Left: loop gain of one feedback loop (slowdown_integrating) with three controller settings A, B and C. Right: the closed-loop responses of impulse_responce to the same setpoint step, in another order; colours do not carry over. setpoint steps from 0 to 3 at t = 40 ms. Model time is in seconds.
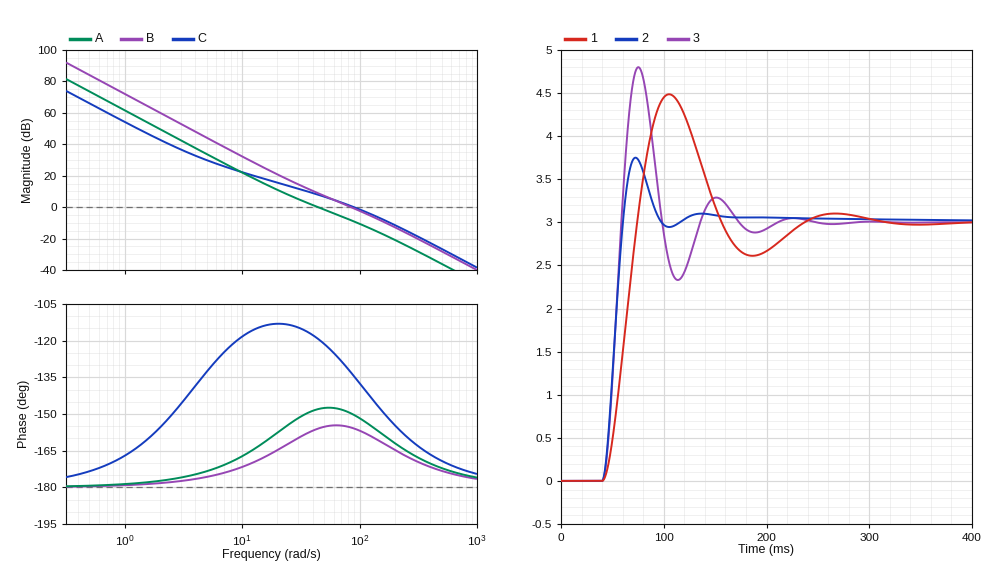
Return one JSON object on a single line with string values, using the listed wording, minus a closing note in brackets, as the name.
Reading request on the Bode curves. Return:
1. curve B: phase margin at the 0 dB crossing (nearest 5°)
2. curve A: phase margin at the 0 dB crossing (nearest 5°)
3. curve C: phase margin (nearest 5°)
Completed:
{"curve B: phase margin at the 0 dB crossing": "25°", "curve A: phase margin at the 0 dB crossing": "30°", "curve C: phase margin": "45°"}
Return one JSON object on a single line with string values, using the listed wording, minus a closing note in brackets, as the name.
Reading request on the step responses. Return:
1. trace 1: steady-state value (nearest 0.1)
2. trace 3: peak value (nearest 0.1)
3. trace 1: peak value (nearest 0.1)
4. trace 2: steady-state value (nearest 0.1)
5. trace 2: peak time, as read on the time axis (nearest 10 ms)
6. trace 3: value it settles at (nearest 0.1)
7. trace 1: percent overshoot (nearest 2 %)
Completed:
{"trace 1: steady-state value": "3.0", "trace 3: peak value": "4.8", "trace 1: peak value": "4.5", "trace 2: steady-state value": "3.0", "trace 2: peak time, as read on the time axis": "70 ms", "trace 3: value it settles at": "3.0", "trace 1: percent overshoot": "50 %"}
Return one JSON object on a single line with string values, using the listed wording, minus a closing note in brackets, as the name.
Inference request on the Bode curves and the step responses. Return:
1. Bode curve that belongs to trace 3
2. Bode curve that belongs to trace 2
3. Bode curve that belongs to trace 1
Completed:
{"Bode curve that belongs to trace 3": "B", "Bode curve that belongs to trace 2": "C", "Bode curve that belongs to trace 1": "A"}
